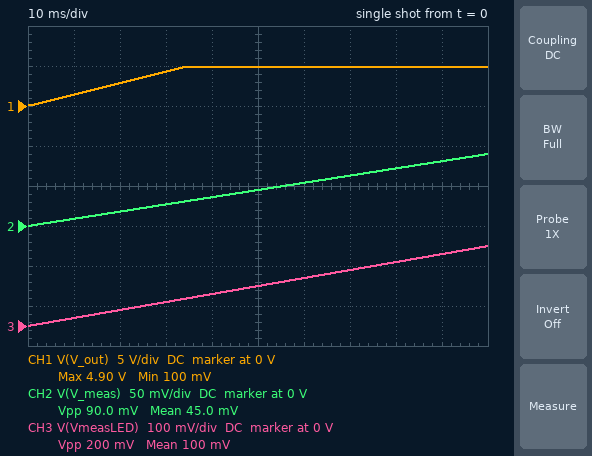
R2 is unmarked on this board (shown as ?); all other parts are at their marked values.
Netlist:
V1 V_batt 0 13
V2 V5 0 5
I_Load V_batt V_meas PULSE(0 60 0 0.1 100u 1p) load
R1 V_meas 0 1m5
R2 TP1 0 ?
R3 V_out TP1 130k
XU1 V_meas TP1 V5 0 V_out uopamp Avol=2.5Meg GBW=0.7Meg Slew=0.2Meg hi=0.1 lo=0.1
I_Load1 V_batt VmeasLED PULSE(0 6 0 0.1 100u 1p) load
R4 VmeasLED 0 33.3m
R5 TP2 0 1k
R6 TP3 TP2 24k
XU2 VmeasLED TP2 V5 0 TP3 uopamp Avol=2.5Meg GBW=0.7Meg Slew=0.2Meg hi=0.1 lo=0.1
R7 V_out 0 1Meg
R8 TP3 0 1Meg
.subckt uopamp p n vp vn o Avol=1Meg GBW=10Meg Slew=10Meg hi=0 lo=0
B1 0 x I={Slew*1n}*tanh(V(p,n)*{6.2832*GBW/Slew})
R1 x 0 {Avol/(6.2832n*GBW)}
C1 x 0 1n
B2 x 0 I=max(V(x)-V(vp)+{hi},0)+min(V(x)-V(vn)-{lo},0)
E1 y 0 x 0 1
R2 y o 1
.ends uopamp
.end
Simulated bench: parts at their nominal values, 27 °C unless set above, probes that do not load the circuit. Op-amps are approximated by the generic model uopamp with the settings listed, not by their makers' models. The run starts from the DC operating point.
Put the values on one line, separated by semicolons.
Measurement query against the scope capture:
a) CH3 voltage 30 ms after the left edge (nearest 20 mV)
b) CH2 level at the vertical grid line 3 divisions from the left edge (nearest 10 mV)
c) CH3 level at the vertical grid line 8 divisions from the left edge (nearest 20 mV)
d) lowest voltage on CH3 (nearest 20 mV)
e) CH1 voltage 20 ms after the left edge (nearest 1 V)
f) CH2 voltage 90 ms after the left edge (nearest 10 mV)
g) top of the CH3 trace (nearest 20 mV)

60 mV; 30 mV; 160 mV; 0 V; 3 V; 80 mV; 200 mV
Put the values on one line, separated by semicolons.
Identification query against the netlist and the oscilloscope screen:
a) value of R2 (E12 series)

820 Ω
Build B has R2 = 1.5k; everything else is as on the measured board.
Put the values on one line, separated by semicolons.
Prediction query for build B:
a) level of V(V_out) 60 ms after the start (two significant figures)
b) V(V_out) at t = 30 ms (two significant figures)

4.7 V; 2.4 V
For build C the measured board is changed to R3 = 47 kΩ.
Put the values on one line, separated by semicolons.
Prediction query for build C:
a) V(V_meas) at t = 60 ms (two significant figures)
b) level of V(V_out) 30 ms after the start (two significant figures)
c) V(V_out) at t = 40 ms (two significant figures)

54 mV; 1.6 V; 2.1 V
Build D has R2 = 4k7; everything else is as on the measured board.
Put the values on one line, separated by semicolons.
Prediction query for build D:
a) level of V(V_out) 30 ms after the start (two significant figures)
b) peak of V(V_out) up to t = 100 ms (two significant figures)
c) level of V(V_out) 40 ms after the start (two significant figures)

770 mV; 2.6 V; 1.0 V
